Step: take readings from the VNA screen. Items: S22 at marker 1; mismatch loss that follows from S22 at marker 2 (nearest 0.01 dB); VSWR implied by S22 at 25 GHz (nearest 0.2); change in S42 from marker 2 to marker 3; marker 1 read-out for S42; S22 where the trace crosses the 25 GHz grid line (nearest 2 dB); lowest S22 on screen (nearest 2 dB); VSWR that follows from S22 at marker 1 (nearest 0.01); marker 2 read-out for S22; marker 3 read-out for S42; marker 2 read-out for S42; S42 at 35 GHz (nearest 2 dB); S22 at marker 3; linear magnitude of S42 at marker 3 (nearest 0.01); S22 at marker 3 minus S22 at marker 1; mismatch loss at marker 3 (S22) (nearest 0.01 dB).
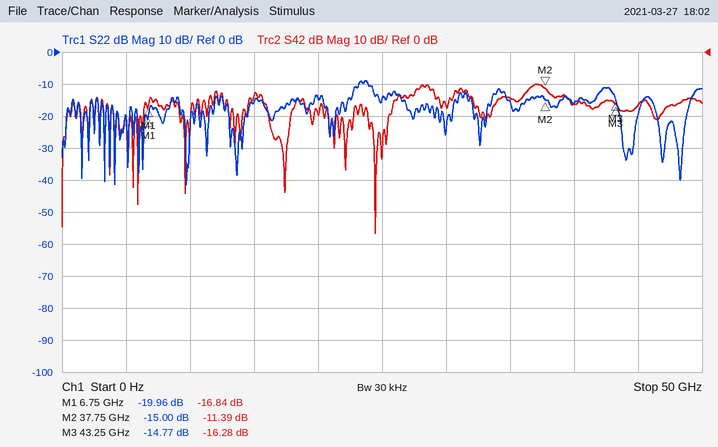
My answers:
-19.96 dB
0.14 dB
1.4
-4.89 dB
-16.84 dB
-14 dB
-42 dB
1.22
-15.00 dB
-16.28 dB
-11.39 dB
-14 dB
-14.77 dB
0.15
5.19 dB
0.15 dB
